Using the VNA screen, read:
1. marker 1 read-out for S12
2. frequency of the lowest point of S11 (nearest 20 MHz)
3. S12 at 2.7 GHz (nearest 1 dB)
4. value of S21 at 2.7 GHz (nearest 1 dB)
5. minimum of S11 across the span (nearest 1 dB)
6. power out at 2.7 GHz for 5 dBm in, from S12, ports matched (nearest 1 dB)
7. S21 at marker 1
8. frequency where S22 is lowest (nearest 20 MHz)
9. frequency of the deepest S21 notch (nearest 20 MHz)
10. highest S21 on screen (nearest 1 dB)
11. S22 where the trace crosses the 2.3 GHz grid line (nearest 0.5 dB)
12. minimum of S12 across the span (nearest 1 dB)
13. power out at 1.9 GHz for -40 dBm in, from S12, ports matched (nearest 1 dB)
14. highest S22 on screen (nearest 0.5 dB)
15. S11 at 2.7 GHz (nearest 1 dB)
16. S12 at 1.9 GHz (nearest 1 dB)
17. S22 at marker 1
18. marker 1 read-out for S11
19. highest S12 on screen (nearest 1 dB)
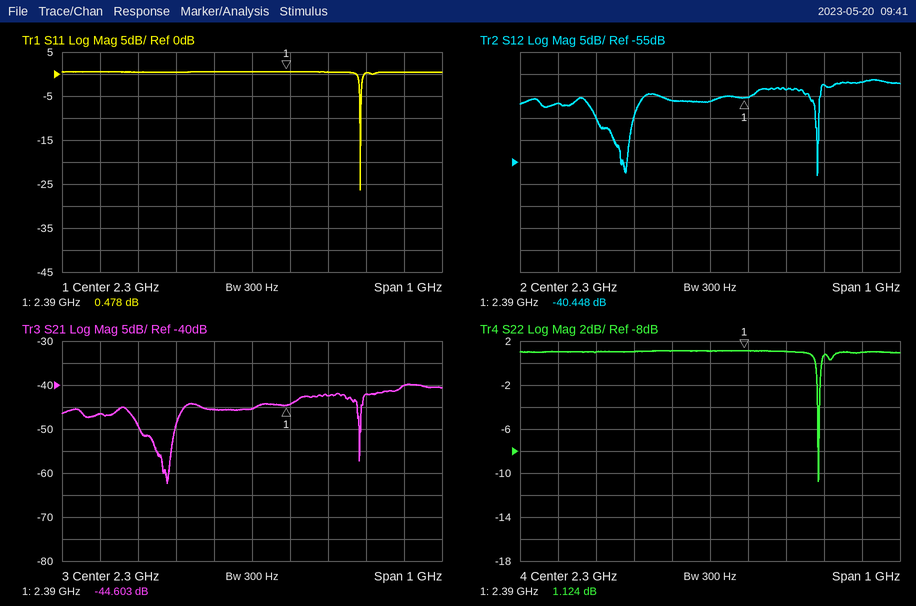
-40.448 dB
2.58 GHz
-37 dB
-40 dB
-26 dB
-32 dBm
-44.603 dB
2.58 GHz
2.08 GHz
-40 dB
1.0 dB
-58 dB
-82 dBm
1.0 dB
0 dB
-42 dB
1.124 dB
0.478 dB
-36 dB
